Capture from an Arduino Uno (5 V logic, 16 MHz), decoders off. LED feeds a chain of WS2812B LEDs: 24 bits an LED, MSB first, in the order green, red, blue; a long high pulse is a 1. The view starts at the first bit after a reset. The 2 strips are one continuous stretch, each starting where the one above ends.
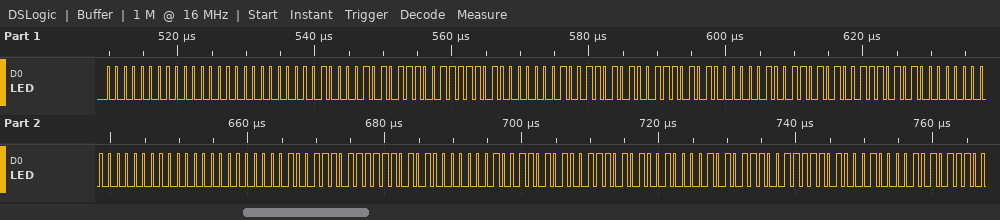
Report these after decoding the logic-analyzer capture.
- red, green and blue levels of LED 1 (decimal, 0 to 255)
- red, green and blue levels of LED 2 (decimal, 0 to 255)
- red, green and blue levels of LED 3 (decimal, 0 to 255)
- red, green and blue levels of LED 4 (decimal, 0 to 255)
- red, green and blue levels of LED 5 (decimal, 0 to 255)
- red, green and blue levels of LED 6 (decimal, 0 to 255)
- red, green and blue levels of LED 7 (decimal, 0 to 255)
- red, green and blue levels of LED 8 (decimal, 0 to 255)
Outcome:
0, 0, 0
185, 66, 244
212, 4, 234
212, 4, 234
0, 0, 0
239, 4, 212
212, 4, 234
185, 66, 244
